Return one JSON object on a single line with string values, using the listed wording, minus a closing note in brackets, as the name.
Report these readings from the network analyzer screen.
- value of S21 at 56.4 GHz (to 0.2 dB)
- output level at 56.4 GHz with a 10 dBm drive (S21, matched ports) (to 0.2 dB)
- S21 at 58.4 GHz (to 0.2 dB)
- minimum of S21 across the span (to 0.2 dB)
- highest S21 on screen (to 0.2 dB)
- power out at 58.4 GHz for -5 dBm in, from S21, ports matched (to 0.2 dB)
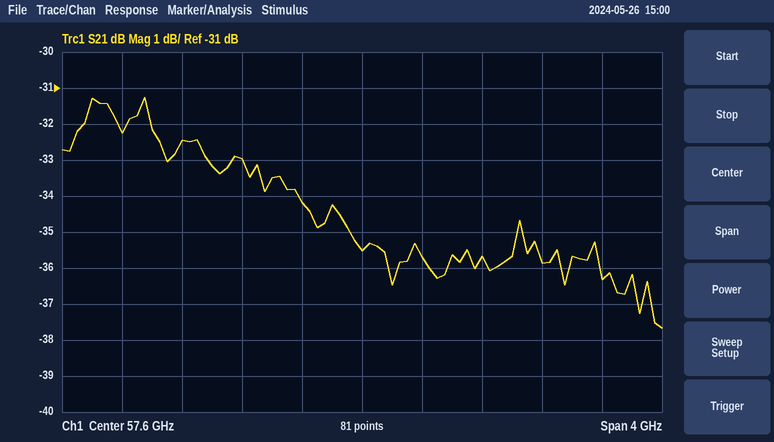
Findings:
{"value of S21 at 56.4 GHz": "-32.4 dB", "output level at 56.4 GHz with a 10 dBm drive (S21, matched ports)": "-22.4 dBm", "S21 at 58.4 GHz": "-35.6 dB", "minimum of S21 across the span": "-37.6 dB", "highest S21 on screen": "-31.2 dB", "power out at 58.4 GHz for -5 dBm in, from S21, ports matched": "-40.6 dBm"}
